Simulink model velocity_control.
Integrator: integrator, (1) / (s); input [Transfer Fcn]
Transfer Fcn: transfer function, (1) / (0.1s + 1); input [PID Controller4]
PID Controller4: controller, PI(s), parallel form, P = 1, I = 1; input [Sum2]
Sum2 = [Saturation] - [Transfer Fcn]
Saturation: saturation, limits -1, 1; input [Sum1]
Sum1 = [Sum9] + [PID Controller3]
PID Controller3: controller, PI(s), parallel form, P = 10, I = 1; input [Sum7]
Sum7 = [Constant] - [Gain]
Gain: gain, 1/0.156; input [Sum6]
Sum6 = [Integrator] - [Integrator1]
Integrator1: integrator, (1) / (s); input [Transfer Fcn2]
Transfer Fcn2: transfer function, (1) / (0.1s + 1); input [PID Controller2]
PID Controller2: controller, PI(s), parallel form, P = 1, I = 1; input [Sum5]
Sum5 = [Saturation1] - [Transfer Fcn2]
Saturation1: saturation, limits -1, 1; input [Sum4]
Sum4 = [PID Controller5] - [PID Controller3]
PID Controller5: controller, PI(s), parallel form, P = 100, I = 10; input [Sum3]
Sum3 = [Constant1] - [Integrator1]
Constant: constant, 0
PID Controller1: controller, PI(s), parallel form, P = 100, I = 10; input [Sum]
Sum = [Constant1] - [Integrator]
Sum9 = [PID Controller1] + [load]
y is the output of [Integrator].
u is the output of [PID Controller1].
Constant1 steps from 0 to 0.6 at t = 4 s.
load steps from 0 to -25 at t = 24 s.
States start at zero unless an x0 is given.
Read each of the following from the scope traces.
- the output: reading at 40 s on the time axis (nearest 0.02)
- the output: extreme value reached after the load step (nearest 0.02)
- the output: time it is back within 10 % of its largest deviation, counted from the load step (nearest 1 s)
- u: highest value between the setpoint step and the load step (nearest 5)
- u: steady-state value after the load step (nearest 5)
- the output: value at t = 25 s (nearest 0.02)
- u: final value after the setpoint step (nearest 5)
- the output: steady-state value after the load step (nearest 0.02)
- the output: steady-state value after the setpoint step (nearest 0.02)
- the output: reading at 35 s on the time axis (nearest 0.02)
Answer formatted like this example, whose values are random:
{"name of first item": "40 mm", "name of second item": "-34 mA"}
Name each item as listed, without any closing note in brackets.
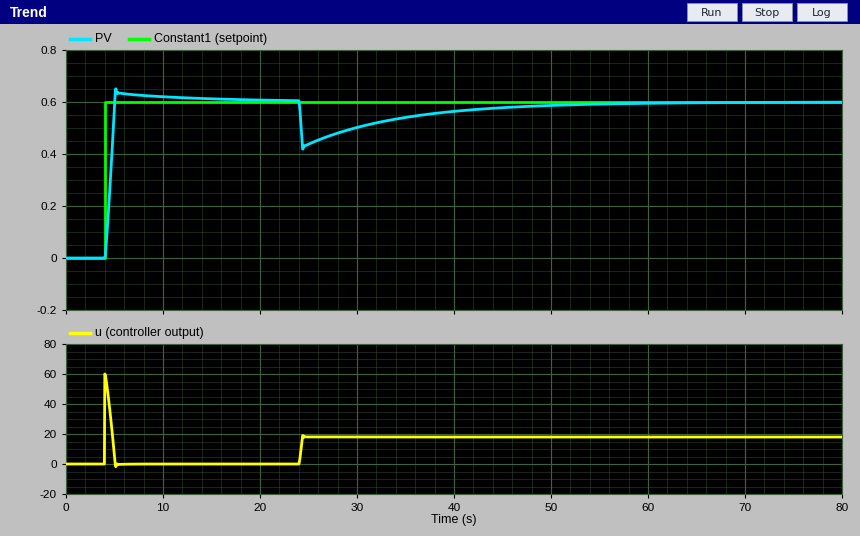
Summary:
{"the output: reading at 40 s on the time axis": "0.56", "the output: extreme value reached after the load step": "0.42", "the output: time it is back within 10 % of its largest deviation, counted from the load step": "23 s", "u: highest value between the setpoint step and the load step": "60", "u: steady-state value after the load step": "20", "the output: value at t = 25 s": "0.44", "u: final value after the setpoint step": "0", "the output: steady-state value after the load step": "0.60", "the output: steady-state value after the setpoint step": "0.60", "the output: reading at 35 s on the time axis": "0.54"}
